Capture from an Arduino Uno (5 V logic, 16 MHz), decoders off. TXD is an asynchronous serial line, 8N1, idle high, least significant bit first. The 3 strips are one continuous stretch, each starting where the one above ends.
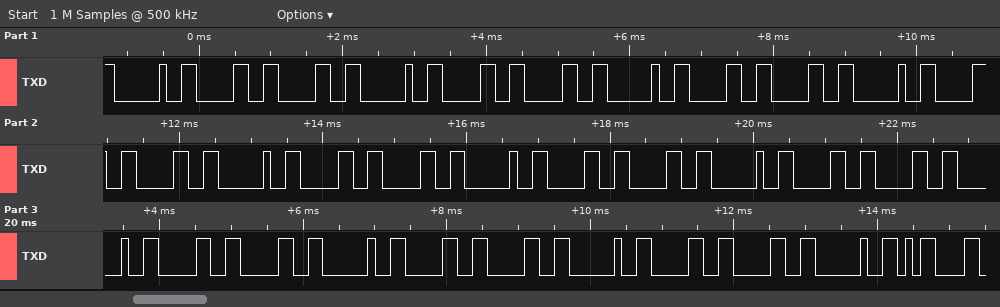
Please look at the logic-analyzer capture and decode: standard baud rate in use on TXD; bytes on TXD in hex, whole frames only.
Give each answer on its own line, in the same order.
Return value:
9600 baud
0x20 0x30 0x30 0x20 0x30 0x30 0x20 0x30 0x30 0x20 0x30 0x30 0x20 0x30 0x30 0x20 0x30 0x30 0x20 0x30 0x30 0x20 0x30 0x30 0x20 0x30 0x30 0x20 0x30 0x30 0x20 0x0D
